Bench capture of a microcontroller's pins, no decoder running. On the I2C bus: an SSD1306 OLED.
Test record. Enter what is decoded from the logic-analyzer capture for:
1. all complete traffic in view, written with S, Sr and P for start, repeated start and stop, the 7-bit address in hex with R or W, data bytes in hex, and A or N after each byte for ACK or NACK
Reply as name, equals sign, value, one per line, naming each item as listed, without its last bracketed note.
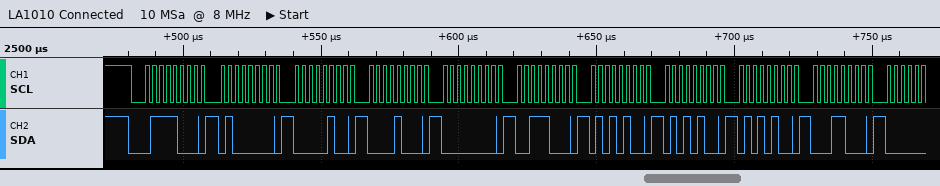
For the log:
all complete traffic in view, written with S, Sr and P for start, repeated start and stop, the 7-bit address in hex with R or W, data bytes in hex, and A or N after each byte for ACK or NACK = S 3CW A 40 A 04 A 08 A 00 A 38 A 54 A 54 A 54 A 18 A
